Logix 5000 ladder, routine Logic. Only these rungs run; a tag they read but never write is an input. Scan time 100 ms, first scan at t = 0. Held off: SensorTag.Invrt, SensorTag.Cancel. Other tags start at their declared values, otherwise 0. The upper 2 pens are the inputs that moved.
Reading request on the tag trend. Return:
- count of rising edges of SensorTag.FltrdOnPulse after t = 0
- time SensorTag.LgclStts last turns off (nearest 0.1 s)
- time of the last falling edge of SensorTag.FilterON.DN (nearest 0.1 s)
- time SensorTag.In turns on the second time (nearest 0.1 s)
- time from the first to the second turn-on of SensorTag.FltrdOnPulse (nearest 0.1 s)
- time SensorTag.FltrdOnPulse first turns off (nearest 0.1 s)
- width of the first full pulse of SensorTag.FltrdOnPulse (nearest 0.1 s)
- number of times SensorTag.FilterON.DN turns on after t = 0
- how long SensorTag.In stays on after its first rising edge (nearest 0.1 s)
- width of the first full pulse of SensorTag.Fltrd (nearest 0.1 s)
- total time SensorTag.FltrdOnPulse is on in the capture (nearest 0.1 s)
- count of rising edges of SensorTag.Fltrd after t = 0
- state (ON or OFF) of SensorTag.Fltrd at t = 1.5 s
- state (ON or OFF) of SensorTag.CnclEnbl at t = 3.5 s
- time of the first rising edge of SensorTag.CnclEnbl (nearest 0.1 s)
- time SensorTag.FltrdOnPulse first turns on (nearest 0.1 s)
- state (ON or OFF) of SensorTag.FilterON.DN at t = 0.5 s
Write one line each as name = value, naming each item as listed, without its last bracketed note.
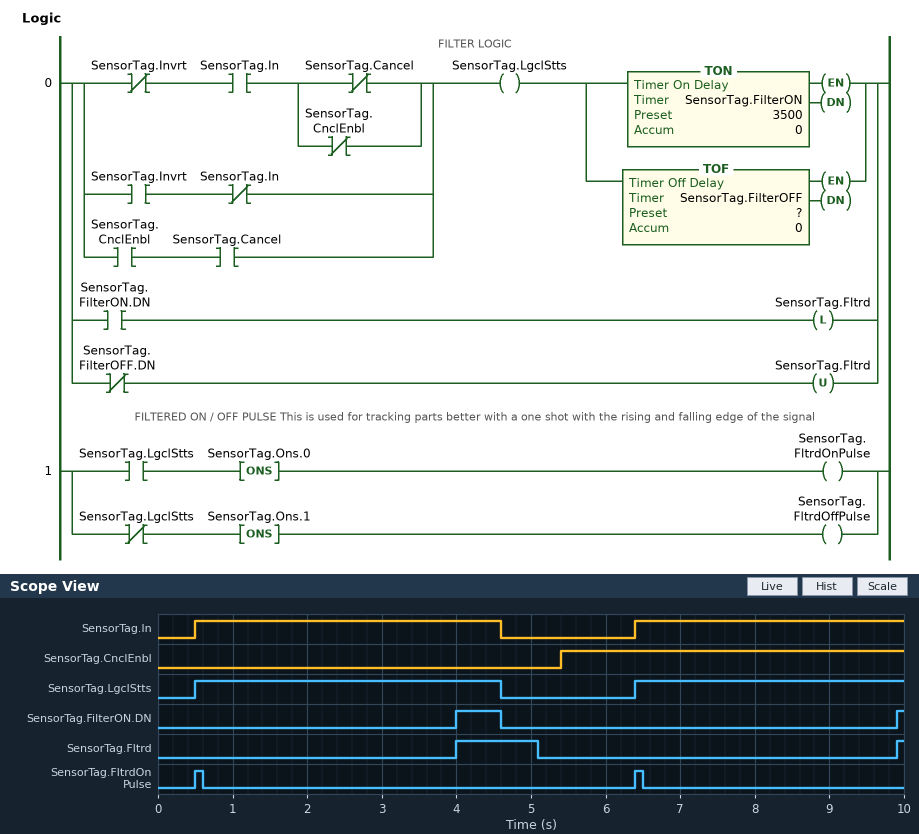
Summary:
count of rising edges of SensorTag.FltrdOnPulse after t = 0 = 2
time SensorTag.LgclStts last turns off = 4.6 s
time of the last falling edge of SensorTag.FilterON.DN = 4.6 s
time SensorTag.In turns on the second time = 6.4 s
time from the first to the second turn-on of SensorTag.FltrdOnPulse = 5.9 s
time SensorTag.FltrdOnPulse first turns off = 0.6 s
width of the first full pulse of SensorTag.FltrdOnPulse = 0.1 s
number of times SensorTag.FilterON.DN turns on after t = 0 = 2
how long SensorTag.In stays on after its first rising edge = 4.1 s
width of the first full pulse of SensorTag.Fltrd = 1.1 s
total time SensorTag.FltrdOnPulse is on in the capture = 0.2 s
count of rising edges of SensorTag.Fltrd after t = 0 = 2
state (ON or OFF) of SensorTag.Fltrd at t = 1.5 s = OFF
state (ON or OFF) of SensorTag.CnclEnbl at t = 3.5 s = OFF
time of the first rising edge of SensorTag.CnclEnbl = 5.4 s
time SensorTag.FltrdOnPulse first turns on = 0.5 s
state (ON or OFF) of SensorTag.FilterON.DN at t = 0.5 s = OFF
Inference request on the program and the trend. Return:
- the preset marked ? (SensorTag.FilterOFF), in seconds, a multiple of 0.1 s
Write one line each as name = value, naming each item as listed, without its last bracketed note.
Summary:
the preset marked ? (SensorTag.FilterOFF), in seconds, a multiple of 0.1 s = 0.5 s
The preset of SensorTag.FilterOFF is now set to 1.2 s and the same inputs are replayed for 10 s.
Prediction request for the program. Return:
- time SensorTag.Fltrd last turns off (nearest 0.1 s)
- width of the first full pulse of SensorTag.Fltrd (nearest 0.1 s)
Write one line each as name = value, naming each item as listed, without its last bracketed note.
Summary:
time SensorTag.Fltrd last turns off = 5.8 s
width of the first full pulse of SensorTag.Fltrd = 1.8 s
